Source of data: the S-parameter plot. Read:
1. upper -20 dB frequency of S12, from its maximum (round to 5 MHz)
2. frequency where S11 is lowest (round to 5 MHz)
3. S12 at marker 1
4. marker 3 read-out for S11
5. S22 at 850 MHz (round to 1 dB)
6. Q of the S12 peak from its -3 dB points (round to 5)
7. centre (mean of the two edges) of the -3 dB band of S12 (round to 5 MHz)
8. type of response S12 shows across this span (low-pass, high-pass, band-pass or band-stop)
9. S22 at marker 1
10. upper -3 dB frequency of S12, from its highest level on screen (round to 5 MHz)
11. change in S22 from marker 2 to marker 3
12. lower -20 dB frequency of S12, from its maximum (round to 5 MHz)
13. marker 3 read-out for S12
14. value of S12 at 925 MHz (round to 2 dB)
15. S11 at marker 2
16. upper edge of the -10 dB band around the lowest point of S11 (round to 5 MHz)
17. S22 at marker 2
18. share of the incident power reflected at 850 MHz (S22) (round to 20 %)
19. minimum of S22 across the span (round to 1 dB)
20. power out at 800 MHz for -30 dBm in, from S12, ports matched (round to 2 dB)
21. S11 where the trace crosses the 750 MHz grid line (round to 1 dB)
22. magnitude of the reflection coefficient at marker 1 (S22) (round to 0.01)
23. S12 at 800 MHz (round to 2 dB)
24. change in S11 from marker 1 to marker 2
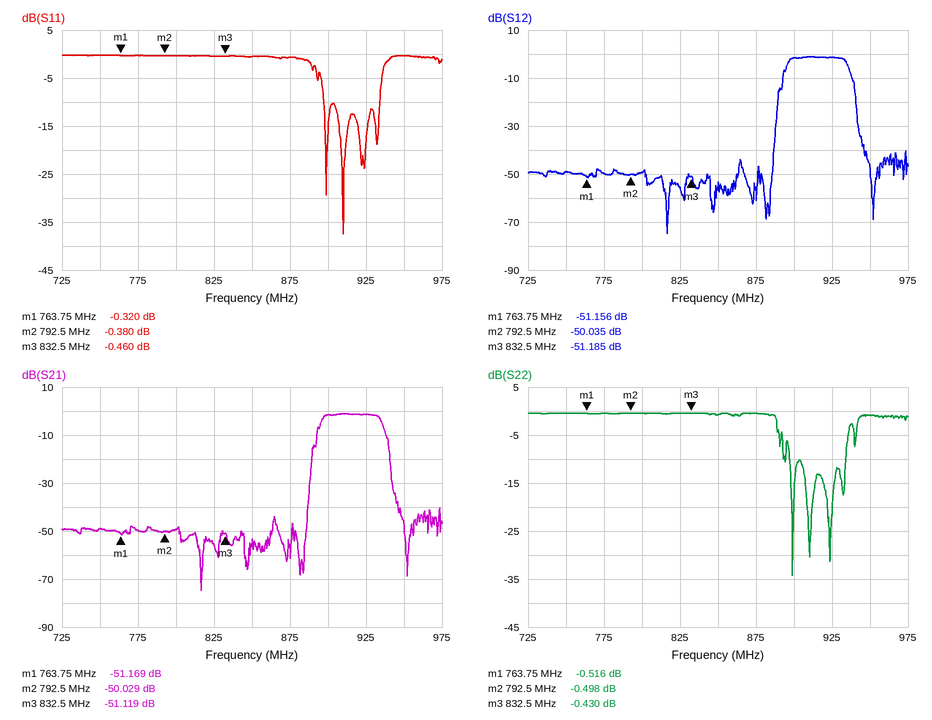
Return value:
940 MHz
910 MHz
-51.156 dB
-0.460 dB
-1 dB
25
915 MHz
band-pass
-0.516 dB
935 MHz
0.068 dB
890 MHz
-51.185 dB
-2 dB
-0.380 dB
935 MHz
-0.498 dB
80 %
-34 dB
-80 dBm
0 dB
0.94
-50 dB
-0.060 dB
